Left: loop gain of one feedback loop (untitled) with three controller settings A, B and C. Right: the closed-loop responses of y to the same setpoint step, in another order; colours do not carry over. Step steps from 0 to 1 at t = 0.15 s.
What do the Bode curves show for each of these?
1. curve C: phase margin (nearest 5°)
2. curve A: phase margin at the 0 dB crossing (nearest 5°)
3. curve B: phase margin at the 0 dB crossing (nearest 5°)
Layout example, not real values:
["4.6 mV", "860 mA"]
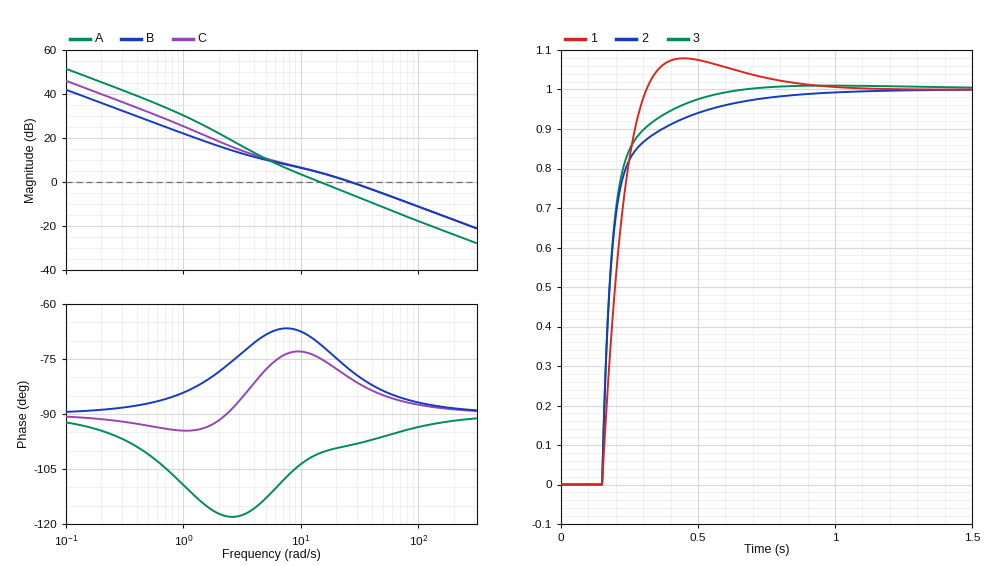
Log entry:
["100°", "80°", "100°"]
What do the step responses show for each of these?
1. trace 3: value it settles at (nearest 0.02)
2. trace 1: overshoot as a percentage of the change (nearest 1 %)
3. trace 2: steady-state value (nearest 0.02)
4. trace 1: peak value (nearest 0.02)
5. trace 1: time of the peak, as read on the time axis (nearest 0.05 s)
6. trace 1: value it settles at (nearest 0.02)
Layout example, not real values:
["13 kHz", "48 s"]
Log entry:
["1.00", "8 %", "1.00", "1.08", "0.45 s", "1.00"]
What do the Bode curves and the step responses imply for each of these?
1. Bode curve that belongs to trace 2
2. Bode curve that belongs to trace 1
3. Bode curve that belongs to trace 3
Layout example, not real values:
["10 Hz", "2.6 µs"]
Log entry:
["B", "A", "C"]
